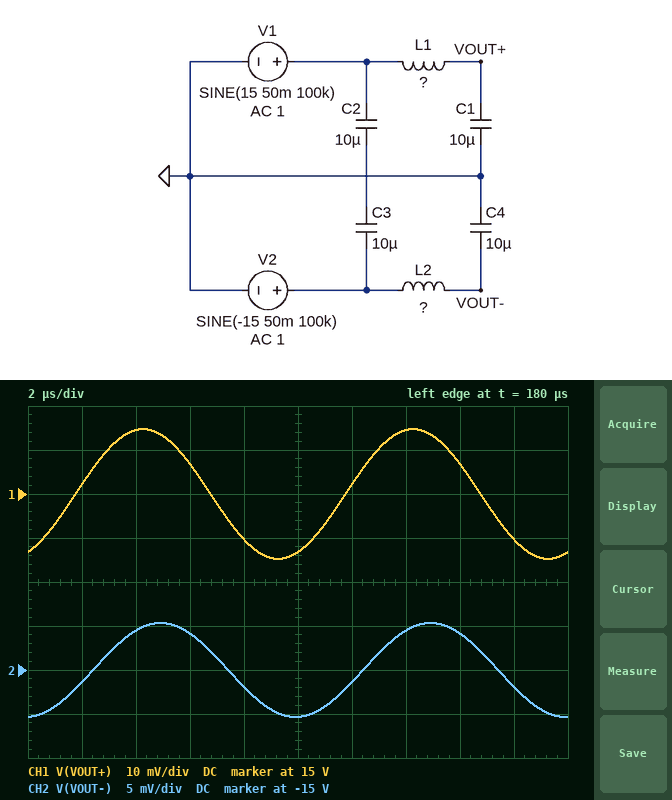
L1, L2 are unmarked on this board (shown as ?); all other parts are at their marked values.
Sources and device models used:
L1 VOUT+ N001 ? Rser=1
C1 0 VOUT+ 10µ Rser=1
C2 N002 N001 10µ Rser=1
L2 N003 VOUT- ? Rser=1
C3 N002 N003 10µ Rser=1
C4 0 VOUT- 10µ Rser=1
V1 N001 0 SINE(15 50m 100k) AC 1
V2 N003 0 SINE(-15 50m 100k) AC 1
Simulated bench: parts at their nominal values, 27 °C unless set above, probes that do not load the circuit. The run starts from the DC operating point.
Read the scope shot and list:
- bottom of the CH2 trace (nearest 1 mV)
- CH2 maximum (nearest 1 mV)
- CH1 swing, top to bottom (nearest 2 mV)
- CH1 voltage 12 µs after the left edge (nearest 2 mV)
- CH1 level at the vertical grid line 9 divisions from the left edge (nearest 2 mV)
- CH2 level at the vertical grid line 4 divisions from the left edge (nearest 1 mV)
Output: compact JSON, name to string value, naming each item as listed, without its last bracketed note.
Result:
{"bottom of the CH2 trace": "-15.005 V", "CH2 maximum": "-14.995 V", "CH1 swing, top to bottom": "30 mV", "CH1 voltage 12 µs after the left edge": "15.002 V", "CH1 level at the vertical grid line 9 divisions from the left edge": "14.990 V", "CH2 level at the vertical grid line 4 divisions from the left edge": "-15.002 V"}
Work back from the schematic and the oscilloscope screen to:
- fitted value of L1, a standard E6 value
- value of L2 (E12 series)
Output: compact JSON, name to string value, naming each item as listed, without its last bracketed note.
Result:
{"fitted value of L1, a standard E6 value": "4.7 µH", "value of L2": "15 µH"}
